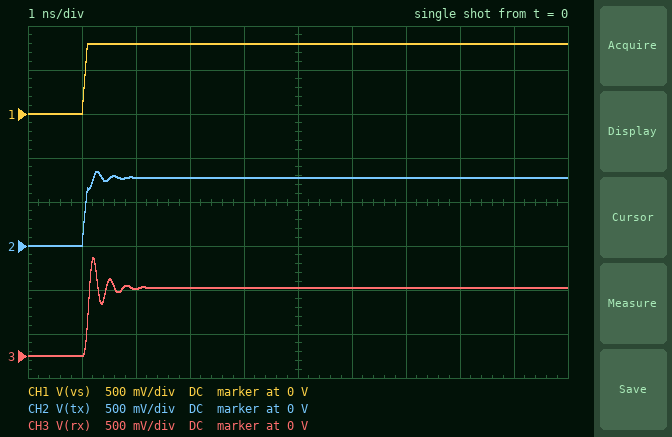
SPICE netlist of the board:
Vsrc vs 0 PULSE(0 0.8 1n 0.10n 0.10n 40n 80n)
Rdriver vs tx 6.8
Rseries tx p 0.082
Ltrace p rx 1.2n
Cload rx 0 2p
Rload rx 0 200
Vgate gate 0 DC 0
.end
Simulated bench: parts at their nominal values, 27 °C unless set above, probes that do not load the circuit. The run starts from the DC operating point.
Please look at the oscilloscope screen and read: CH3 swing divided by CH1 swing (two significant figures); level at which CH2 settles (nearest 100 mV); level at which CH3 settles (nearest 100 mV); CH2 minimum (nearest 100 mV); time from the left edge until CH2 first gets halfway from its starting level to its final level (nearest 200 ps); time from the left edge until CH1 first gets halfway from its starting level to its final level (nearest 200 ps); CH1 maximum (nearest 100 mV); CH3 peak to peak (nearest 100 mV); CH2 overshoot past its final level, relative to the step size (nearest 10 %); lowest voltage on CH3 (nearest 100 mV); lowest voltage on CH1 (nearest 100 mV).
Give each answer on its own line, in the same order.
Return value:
1.4
800 mV
800 mV
0 V
1.0 ns
1.0 ns
800 mV
1.1 V
10 %
0 V
0 V
